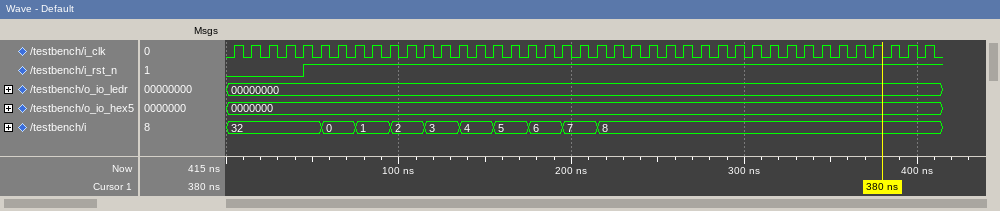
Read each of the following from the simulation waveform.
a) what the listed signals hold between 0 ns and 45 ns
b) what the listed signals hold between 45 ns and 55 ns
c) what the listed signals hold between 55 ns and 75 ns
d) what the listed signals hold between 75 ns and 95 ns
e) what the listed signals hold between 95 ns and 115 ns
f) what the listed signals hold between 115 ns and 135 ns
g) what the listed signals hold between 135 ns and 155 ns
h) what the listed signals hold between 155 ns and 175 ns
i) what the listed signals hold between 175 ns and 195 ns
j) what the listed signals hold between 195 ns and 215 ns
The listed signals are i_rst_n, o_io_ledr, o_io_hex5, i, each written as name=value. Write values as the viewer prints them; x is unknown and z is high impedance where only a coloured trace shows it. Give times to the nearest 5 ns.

i_rst_n=0, o_io_ledr=00000000, o_io_hex5=0000000, i=32
i_rst_n=1, o_io_ledr=00000000, o_io_hex5=0000000, i=32
i_rst_n=1, o_io_ledr=00000000, o_io_hex5=0000000, i=0
i_rst_n=1, o_io_ledr=00000000, o_io_hex5=0000000, i=1
i_rst_n=1, o_io_ledr=00000000, o_io_hex5=0000000, i=2
i_rst_n=1, o_io_ledr=00000000, o_io_hex5=0000000, i=3
i_rst_n=1, o_io_ledr=00000000, o_io_hex5=0000000, i=4
i_rst_n=1, o_io_ledr=00000000, o_io_hex5=0000000, i=5
i_rst_n=1, o_io_ledr=00000000, o_io_hex5=0000000, i=6
i_rst_n=1, o_io_ledr=00000000, o_io_hex5=0000000, i=7
